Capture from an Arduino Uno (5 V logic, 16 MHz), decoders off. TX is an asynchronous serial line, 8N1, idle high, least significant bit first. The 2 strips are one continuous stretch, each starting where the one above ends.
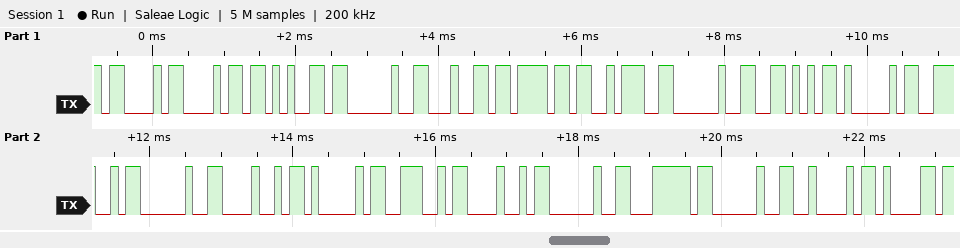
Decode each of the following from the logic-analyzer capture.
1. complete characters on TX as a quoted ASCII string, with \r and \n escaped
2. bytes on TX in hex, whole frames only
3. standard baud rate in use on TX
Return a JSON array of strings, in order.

["\"Che do: VAN HANH | Ba\"", "43 68 65 20 64 6F 3A 20 56 41 4E 20 48 41 4E 48 20 7C 20 42 61", "9600 baud"]
